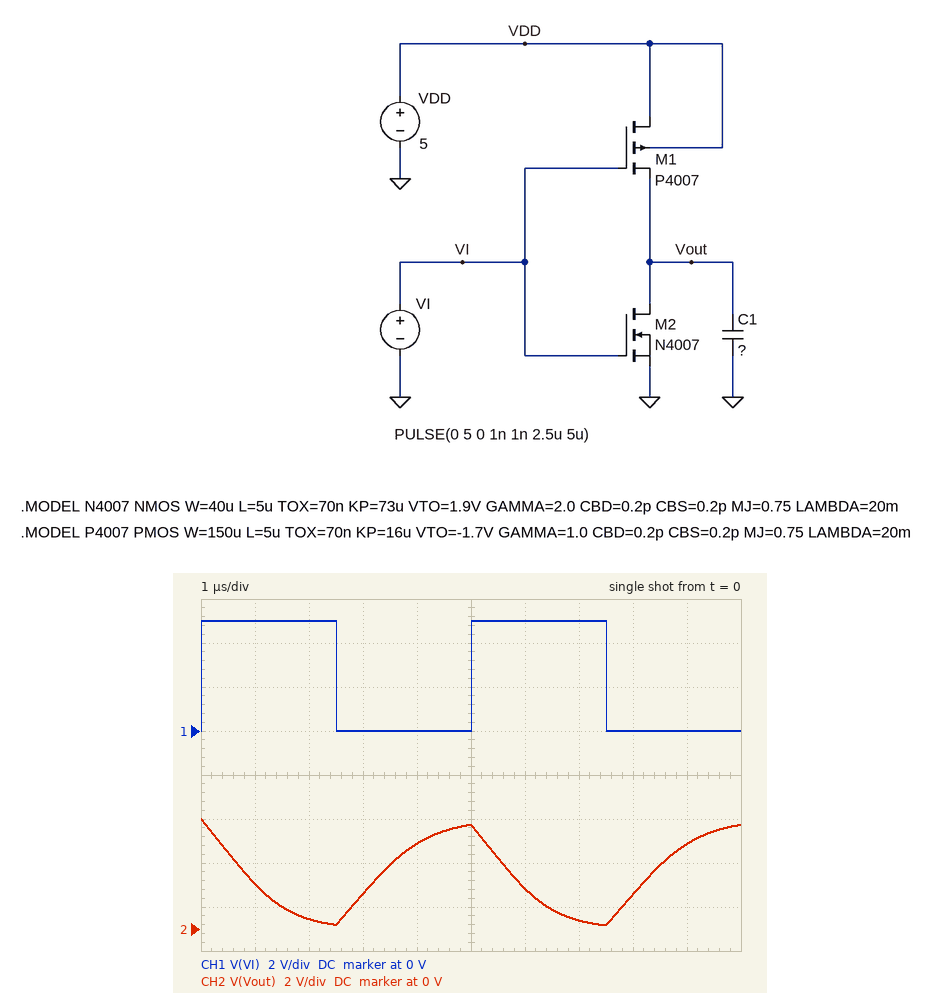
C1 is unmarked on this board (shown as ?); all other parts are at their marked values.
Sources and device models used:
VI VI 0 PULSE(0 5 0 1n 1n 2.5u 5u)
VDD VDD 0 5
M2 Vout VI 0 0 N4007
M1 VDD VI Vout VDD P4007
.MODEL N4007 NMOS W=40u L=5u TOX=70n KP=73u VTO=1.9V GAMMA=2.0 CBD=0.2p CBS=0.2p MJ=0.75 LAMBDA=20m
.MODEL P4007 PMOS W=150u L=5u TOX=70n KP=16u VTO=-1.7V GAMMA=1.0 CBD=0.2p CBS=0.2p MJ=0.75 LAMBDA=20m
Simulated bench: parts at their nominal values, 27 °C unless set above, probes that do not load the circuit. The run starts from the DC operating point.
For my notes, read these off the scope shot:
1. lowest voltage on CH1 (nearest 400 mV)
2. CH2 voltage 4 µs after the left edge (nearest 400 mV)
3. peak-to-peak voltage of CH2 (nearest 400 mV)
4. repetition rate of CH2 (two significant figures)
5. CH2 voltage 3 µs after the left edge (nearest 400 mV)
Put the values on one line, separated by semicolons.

0 V; 4.0 V; 4.8 V; 200 kHz; 1.6 V
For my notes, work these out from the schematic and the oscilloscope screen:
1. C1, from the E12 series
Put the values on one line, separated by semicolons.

1 nF
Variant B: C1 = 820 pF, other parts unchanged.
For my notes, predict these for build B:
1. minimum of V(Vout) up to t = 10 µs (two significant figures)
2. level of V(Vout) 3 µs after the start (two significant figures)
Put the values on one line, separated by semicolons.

66 mV; 1.8 V
